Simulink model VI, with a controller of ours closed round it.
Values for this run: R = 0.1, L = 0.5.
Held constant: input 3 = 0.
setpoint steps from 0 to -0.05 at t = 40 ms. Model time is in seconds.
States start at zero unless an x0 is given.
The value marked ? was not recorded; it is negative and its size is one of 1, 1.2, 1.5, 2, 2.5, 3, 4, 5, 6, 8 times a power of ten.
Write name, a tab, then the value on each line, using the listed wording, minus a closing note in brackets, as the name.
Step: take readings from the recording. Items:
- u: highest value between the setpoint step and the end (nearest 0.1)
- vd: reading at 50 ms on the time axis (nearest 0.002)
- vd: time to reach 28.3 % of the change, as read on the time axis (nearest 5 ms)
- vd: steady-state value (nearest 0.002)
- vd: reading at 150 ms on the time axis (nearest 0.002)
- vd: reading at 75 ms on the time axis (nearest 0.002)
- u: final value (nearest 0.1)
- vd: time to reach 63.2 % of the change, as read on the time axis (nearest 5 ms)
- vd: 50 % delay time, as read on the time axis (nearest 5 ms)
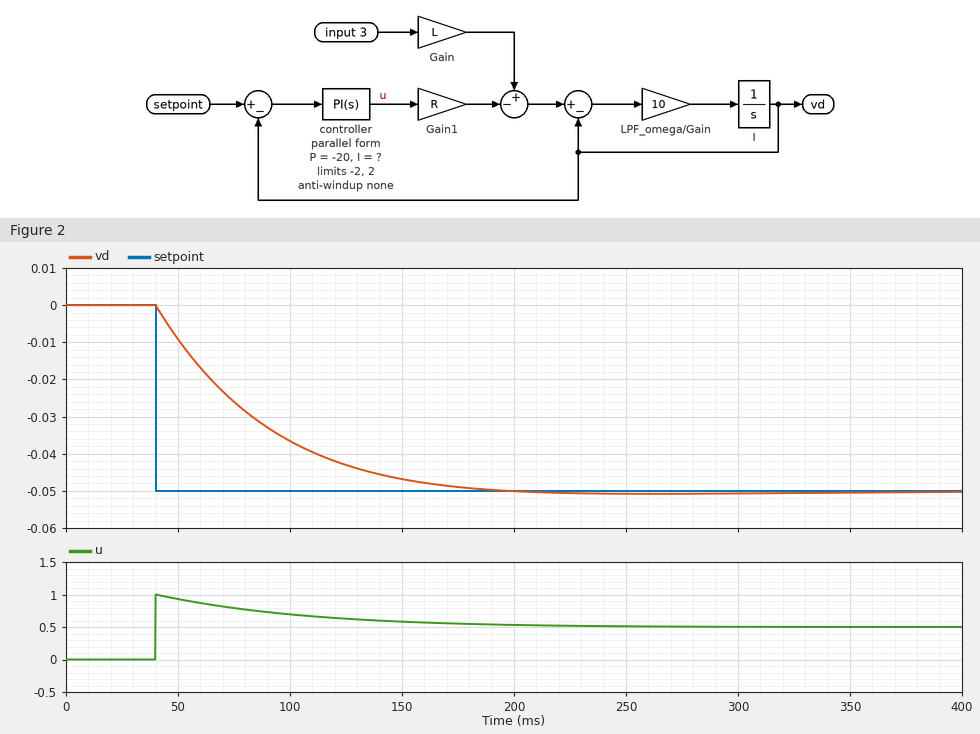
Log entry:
u: highest value between the setpoint step and the end	1.0
vd: reading at 50 ms on the time axis	-0.010
vd: time to reach 28.3 % of the change, as read on the time axis	55 ms
vd: steady-state value	-0.050
vd: reading at 150 ms on the time axis	-0.046
vd: reading at 75 ms on the time axis	-0.026
u: final value	0.5
vd: time to reach 63.2 % of the change, as read on the time axis	85 ms
vd: 50 % delay time, as read on the time axis	75 ms
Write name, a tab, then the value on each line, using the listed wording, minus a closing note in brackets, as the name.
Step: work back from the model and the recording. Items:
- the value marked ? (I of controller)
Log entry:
the value marked ?	-250
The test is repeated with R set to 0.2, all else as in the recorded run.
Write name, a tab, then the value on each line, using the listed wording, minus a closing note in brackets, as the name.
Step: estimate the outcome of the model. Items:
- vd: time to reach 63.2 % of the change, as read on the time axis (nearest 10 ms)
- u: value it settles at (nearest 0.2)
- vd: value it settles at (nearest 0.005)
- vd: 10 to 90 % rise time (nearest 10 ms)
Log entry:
vd: time to reach 63.2 % of the change, as read on the time axis	60 ms
u: value it settles at	0.2
vd: value it settles at	-0.050
vd: 10 to 90 % rise time	50 ms
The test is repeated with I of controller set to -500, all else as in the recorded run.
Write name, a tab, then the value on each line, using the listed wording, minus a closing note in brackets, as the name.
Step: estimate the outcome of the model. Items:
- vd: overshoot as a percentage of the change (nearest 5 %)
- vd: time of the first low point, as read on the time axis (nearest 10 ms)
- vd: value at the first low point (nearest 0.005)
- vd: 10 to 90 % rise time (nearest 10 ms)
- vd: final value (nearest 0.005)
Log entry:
vd: overshoot as a percentage of the change	10 %
vd: time of the first low point, as read on the time axis	170 ms
vd: value at the first low point	-0.055
vd: 10 to 90 % rise time	60 ms
vd: final value	-0.050
